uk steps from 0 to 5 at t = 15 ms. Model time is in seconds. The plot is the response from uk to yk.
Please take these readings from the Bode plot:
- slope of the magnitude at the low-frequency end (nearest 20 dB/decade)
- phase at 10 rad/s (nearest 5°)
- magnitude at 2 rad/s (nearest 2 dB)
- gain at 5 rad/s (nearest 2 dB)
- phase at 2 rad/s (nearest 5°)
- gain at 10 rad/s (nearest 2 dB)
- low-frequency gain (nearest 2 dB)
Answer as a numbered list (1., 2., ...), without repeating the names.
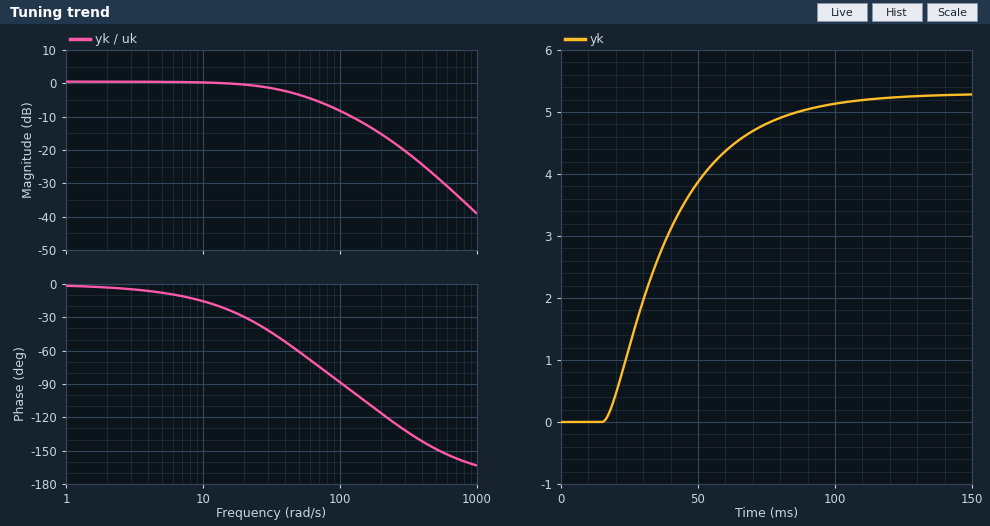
1. 0 dB/decade
2. -15°
3. 0 dB
4. 0 dB
5. -5°
6. 0 dB
7. 0 dB
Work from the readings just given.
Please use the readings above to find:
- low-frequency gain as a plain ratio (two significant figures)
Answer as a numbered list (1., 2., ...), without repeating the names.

1. 1.0
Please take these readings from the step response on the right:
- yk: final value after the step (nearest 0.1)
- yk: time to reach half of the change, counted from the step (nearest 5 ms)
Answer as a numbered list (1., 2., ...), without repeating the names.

1. 5.3
2. 20 ms
